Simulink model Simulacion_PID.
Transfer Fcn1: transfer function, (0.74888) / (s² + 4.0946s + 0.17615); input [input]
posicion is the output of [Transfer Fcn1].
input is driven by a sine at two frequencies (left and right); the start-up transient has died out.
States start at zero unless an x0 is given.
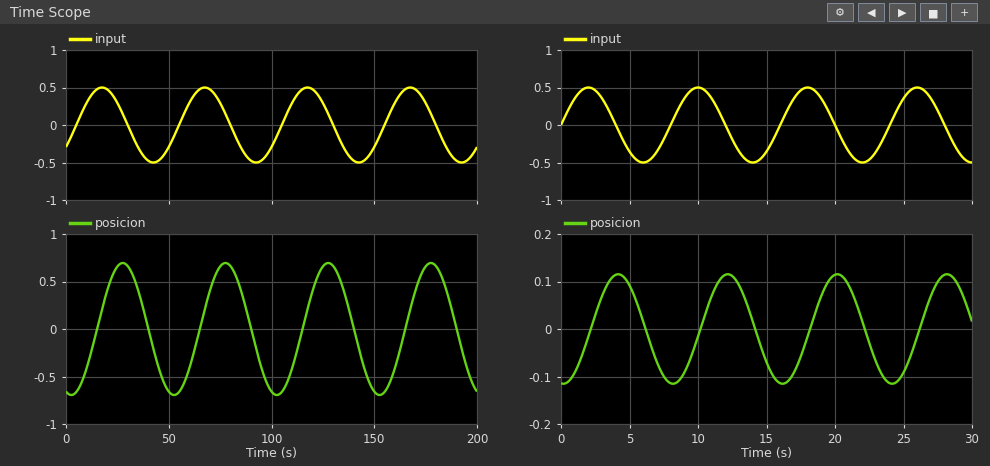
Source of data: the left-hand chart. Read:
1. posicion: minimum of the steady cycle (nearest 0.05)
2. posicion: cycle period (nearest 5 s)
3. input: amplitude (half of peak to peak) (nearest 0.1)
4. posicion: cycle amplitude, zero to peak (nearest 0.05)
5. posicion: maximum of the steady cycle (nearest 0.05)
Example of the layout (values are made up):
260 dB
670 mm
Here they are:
-0.70
50 s
0.5
0.70
0.70
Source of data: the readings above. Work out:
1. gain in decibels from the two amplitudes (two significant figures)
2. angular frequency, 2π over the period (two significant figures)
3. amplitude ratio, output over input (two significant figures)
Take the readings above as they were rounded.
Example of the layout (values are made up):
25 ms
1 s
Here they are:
2.9 dB
0.13 rad/s
1.4
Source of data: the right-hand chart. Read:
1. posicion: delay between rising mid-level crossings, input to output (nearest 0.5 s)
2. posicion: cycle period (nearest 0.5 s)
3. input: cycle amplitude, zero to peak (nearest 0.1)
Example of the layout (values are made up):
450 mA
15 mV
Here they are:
2.0 s
8.0 s
0.5
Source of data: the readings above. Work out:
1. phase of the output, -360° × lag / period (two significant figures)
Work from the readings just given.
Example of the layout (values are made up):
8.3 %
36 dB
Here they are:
-90°
